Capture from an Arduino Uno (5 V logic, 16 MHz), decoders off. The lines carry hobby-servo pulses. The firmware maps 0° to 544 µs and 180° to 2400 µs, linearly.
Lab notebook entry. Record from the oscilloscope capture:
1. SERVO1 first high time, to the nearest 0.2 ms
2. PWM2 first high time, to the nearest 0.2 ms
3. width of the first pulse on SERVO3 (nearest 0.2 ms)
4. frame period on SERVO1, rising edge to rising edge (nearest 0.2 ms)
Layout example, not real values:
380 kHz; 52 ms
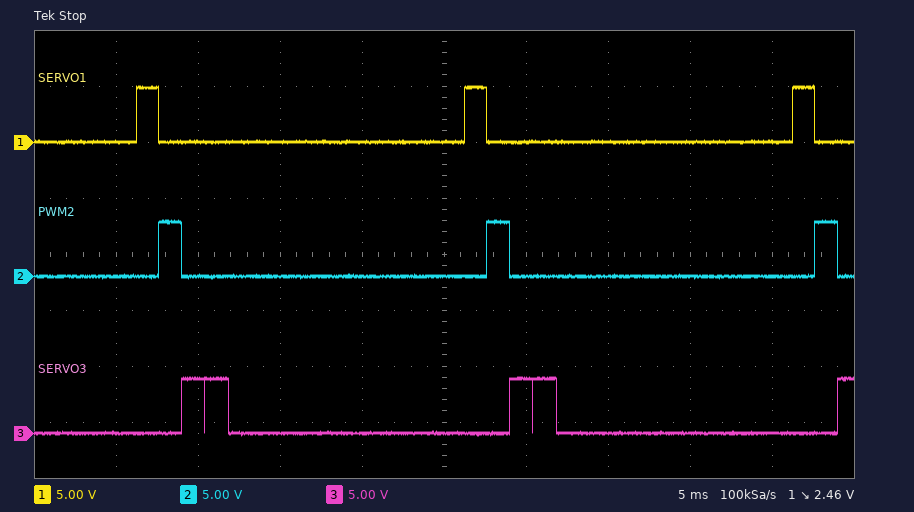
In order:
1.4 ms; 1.4 ms; 1.4 ms; 20.0 ms
